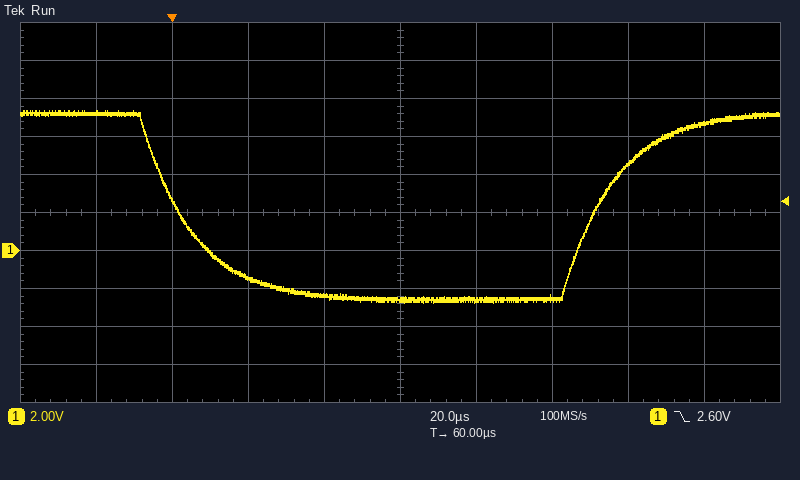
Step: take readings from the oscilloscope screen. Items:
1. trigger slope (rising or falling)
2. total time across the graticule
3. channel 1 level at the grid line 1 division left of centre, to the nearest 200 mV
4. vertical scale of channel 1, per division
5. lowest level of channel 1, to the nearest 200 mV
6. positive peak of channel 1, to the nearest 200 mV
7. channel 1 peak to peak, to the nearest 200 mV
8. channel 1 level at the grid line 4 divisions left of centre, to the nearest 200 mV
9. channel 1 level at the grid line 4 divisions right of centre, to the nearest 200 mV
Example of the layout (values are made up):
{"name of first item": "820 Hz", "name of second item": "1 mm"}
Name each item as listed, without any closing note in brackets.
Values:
{"trigger slope": "falling", "total time across the graticule": "200 µs", "channel 1 level at the grid line 1 division left of centre, to the nearest 200 mV": "-2.4 V", "vertical scale of channel 1, per division": "2 V", "lowest level of channel 1, to the nearest 200 mV": "-2.8 V", "positive peak of channel 1, to the nearest 200 mV": "7.4 V", "channel 1 peak to peak, to the nearest 200 mV": "10.2 V", "channel 1 level at the grid line 4 divisions left of centre, to the nearest 200 mV": "7.2 V", "channel 1 level at the grid line 4 divisions right of centre, to the nearest 200 mV": "6.6 V"}
